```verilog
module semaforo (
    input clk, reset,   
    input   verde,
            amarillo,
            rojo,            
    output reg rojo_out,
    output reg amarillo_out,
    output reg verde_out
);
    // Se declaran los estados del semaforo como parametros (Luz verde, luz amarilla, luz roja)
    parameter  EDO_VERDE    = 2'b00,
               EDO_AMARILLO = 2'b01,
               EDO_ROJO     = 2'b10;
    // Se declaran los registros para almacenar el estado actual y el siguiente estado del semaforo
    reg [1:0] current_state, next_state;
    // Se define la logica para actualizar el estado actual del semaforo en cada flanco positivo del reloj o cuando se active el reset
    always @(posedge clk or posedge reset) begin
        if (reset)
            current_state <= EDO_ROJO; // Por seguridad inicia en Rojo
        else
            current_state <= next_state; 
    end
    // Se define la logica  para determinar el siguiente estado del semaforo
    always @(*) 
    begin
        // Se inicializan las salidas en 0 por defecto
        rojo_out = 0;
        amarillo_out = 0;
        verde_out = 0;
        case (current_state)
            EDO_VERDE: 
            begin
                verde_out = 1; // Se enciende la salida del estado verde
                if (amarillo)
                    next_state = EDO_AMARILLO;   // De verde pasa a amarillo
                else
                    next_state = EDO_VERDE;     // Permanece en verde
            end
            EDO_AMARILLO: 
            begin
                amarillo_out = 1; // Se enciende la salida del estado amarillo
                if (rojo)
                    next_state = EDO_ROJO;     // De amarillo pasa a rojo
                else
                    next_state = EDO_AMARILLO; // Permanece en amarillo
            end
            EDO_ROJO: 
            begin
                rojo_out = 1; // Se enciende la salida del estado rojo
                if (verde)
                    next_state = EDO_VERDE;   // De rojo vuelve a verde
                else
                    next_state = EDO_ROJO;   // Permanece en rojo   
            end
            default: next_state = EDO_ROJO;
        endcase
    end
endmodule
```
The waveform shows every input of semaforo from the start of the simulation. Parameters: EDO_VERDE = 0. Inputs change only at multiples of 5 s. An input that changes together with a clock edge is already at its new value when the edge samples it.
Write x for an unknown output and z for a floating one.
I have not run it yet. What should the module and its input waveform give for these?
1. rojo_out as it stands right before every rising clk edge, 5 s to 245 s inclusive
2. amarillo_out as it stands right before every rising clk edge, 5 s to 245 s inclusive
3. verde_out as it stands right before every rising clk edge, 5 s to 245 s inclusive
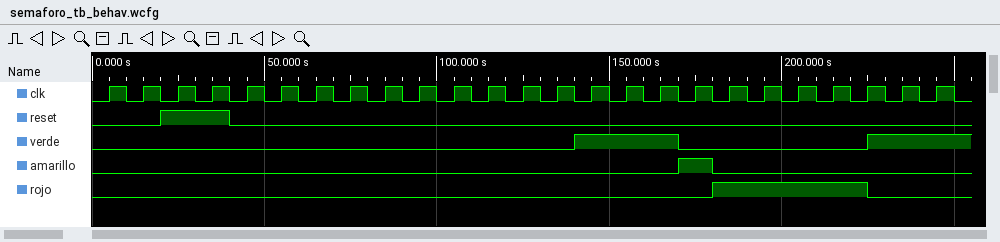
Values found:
0 1 1 1 1 1 1 1 1 1 1 1 1 1 1 0 0 0 0 1 1 1 1 0 0
0 0 0 0 0 0 0 0 0 0 0 0 0 0 0 0 0 0 1 0 0 0 0 0 0
0 0 0 0 0 0 0 0 0 0 0 0 0 0 0 1 1 1 0 0 0 0 0 1 1
